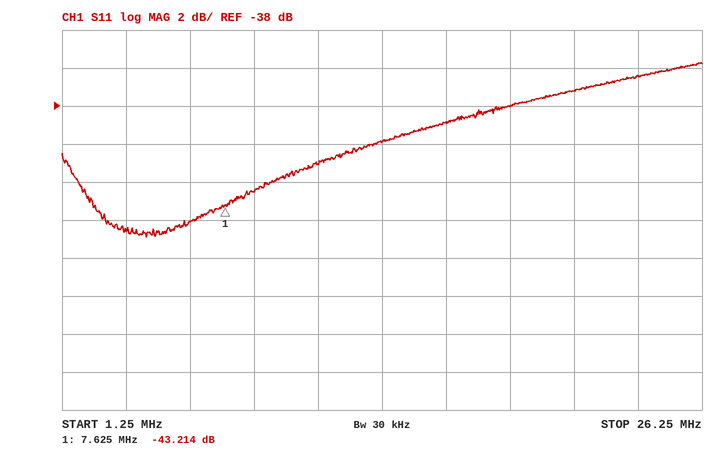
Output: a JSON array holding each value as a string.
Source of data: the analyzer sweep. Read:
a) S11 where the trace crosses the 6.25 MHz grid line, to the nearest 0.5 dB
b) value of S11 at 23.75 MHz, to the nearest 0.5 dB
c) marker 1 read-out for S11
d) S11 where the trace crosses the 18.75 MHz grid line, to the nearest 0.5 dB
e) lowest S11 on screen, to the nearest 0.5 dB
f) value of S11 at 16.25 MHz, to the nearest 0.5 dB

["-44.0 dB", "-36.5 dB", "-43.214 dB", "-38.0 dB", "-45.0 dB", "-39.0 dB"]
